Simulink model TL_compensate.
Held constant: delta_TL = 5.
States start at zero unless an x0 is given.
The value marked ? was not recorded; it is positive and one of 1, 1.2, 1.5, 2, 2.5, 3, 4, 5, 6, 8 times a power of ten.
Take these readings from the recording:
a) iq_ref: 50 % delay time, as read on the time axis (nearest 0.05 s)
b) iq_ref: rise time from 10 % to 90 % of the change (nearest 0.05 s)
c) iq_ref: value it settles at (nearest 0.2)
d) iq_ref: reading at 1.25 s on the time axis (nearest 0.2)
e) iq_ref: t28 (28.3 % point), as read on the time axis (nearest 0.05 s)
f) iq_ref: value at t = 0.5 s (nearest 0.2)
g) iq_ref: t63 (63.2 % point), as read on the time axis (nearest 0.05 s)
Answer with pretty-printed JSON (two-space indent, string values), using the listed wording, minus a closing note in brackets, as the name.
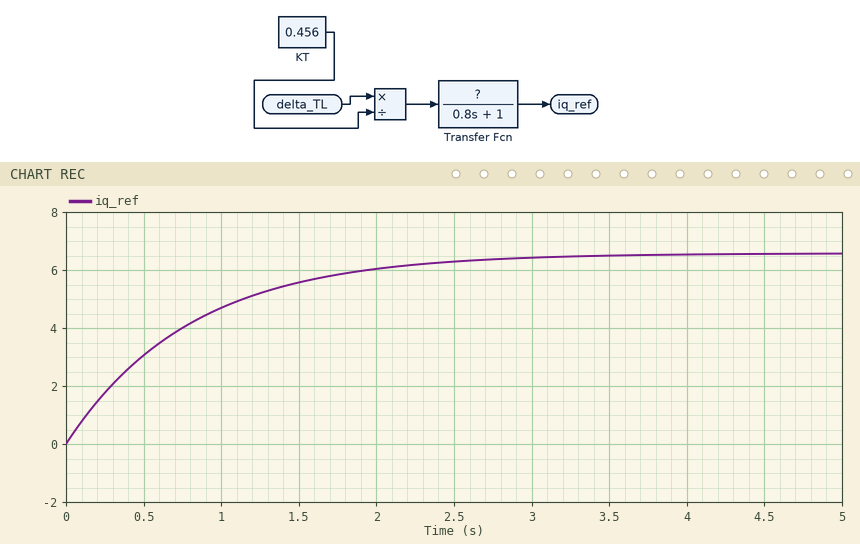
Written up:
{
  "iq_ref: 50 % delay time, as read on the time axis": "0.55 s",
  "iq_ref: rise time from 10 % to 90 % of the change": "1.75 s",
  "iq_ref: value it settles at": "6.6",
  "iq_ref: reading at 1.25 s on the time axis": "5.2",
  "iq_ref: t28 (28.3 % point), as read on the time axis": "0.25 s",
  "iq_ref: value at t = 0.5 s": "3.0",
  "iq_ref: t63 (63.2 % point), as read on the time axis": "0.80 s"
}
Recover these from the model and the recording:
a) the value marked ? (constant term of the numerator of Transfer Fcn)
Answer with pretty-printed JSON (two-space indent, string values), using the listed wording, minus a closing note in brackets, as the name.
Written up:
{
  "the value marked ?": "0.6"
}
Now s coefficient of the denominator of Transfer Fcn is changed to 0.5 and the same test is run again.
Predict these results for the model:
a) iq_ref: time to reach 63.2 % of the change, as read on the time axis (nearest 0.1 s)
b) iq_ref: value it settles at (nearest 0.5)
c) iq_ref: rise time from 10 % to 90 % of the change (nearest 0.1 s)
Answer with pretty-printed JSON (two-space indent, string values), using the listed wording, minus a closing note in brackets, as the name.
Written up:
{
  "iq_ref: time to reach 63.2 % of the change, as read on the time axis": "0.5 s",
  "iq_ref: value it settles at": "6.5",
  "iq_ref: rise time from 10 % to 90 % of the change": "1.1 s"
}
